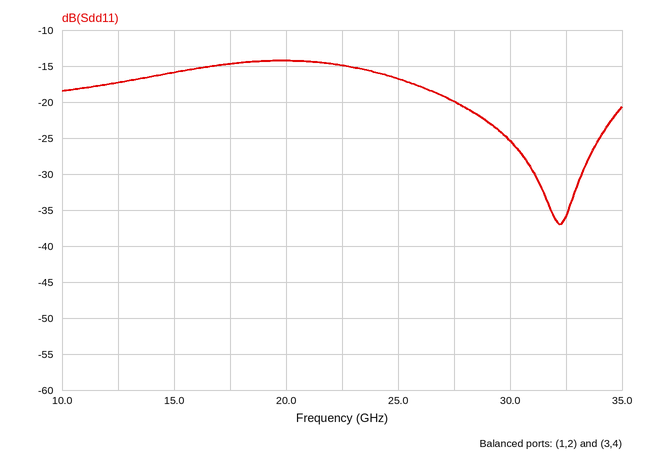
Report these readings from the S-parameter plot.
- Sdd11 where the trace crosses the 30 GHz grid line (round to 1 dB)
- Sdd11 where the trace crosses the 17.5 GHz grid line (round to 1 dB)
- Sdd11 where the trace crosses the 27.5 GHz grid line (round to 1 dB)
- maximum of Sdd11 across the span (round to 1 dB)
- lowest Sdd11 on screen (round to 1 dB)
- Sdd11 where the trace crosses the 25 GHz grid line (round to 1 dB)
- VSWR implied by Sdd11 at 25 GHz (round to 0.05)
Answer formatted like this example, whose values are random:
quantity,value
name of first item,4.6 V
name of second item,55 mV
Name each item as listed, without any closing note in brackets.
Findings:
quantity,value
Sdd11 where the trace crosses the 30 GHz grid line,-25 dB
Sdd11 where the trace crosses the 17.5 GHz grid line,-15 dB
Sdd11 where the trace crosses the 27.5 GHz grid line,-20 dB
maximum of Sdd11 across the span,-14 dB
lowest Sdd11 on screen,-37 dB
Sdd11 where the trace crosses the 25 GHz grid line,-17 dB
VSWR implied by Sdd11 at 25 GHz,1.35
